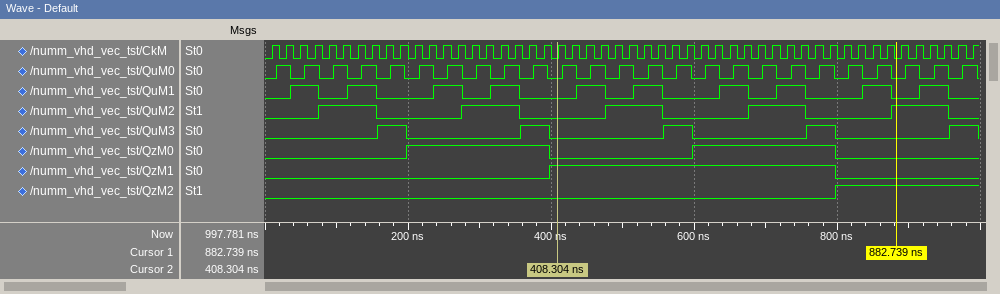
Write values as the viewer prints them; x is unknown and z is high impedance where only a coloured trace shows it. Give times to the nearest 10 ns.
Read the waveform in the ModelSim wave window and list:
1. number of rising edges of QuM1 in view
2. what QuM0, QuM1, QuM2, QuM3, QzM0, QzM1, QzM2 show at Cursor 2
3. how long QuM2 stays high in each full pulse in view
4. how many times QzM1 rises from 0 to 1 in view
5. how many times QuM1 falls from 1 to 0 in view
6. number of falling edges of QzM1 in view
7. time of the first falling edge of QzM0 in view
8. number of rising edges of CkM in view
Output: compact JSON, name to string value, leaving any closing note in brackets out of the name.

{"number of rising edges of QuM1 in view": "10", "what QuM0, QuM1, QuM2, QuM3, QzM0, QzM1, QzM2 show at Cursor 2": "QuM0=0, QuM1=0, QuM2=0, QuM3=0, QzM0=0, QzM1=1, QzM2=0", "how long QuM2 stays high in each full pulse in view": "80 ns, 80 ns, 80 ns, 80 ns, 80 ns", "how many times QzM1 rises from 0 to 1 in view": "1", "how many times QuM1 falls from 1 to 0 in view": "10", "number of falling edges of QzM1 in view": "1", "time of the first falling edge of QzM0 in view": "400 ns", "number of rising edges of CkM in view": "50"}
